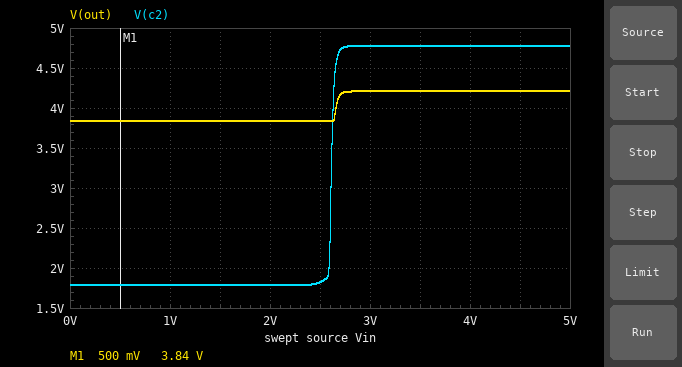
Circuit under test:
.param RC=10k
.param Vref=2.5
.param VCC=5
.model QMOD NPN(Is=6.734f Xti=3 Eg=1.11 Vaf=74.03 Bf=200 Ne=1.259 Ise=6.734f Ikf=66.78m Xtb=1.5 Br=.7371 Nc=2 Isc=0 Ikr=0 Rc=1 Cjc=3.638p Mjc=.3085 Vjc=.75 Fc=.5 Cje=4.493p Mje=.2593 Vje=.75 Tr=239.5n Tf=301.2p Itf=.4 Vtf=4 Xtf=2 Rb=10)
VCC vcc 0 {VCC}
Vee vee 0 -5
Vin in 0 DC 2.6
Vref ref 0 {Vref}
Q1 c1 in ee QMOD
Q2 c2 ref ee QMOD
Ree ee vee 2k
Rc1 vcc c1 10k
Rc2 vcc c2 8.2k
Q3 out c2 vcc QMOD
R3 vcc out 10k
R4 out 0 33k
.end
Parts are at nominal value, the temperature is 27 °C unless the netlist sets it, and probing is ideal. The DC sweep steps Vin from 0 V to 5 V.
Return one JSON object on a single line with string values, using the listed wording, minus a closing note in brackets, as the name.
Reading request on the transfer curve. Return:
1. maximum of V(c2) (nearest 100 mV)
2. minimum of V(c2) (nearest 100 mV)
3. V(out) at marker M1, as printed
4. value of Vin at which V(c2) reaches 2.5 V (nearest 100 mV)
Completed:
{"maximum of V(c2)": "4.8 V", "minimum of V(c2)": "1.8 V", "V(out) at marker M1, as printed": "3.84 V", "value of Vin at which V(c2) reaches 2.5 V": "2.6 V"}
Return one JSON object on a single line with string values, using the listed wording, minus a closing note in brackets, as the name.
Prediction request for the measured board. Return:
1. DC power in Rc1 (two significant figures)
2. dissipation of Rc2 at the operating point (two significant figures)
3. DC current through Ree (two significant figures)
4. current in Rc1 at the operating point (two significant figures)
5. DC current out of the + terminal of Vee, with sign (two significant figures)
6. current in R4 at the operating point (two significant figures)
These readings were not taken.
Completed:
{"DC power in Rc1": "970 µW", "dissipation of Rc2 at the operating point": "870 µW", "DC current through Ree": "3.4 mA", "current in Rc1 at the operating point": "310 µA", "DC current out of the + terminal of Vee, with sign": "-3.4 mA", "current in R4 at the operating point": "120 µA"}
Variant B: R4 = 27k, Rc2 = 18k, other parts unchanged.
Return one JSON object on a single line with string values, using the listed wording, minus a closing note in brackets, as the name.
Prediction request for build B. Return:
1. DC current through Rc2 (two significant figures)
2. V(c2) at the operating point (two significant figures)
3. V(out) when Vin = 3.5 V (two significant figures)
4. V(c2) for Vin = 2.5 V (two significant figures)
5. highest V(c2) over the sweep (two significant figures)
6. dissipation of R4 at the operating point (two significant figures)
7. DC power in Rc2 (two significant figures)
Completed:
{"DC current through Rc2": "170 µA", "V(c2) at the operating point": "1.9 V", "V(out) when Vin = 3.5 V": "4.0 V", "V(c2) for Vin = 2.5 V": "1.8 V", "highest V(c2) over the sweep": "4.5 V", "dissipation of R4 at the operating point": "490 µW", "DC power in Rc2": "530 µW"}
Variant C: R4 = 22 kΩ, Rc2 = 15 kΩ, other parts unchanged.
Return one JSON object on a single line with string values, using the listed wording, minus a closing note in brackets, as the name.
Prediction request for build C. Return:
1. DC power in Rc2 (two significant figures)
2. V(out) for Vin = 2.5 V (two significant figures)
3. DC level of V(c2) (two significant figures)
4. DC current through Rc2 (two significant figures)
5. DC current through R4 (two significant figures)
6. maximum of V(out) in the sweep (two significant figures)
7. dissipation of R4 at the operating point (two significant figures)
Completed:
{"DC power in Rc2": "640 µW", "V(out) for Vin = 2.5 V": "3.4 V", "DC level of V(c2)": "1.9 V", "DC current through Rc2": "210 µA", "DC current through R4": "160 µA", "maximum of V(out) in the sweep": "3.9 V", "dissipation of R4 at the operating point": "540 µW"}
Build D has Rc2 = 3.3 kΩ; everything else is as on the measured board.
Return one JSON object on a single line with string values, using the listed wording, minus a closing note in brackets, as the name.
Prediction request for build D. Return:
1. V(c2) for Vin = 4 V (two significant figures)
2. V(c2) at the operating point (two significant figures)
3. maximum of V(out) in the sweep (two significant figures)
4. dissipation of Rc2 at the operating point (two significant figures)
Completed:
{"V(c2) for Vin = 4 V": "4.9 V", "V(c2) at the operating point": "3.9 V", "maximum of V(out) in the sweep": "4.3 V", "dissipation of Rc2 at the operating point": "360 µW"}
